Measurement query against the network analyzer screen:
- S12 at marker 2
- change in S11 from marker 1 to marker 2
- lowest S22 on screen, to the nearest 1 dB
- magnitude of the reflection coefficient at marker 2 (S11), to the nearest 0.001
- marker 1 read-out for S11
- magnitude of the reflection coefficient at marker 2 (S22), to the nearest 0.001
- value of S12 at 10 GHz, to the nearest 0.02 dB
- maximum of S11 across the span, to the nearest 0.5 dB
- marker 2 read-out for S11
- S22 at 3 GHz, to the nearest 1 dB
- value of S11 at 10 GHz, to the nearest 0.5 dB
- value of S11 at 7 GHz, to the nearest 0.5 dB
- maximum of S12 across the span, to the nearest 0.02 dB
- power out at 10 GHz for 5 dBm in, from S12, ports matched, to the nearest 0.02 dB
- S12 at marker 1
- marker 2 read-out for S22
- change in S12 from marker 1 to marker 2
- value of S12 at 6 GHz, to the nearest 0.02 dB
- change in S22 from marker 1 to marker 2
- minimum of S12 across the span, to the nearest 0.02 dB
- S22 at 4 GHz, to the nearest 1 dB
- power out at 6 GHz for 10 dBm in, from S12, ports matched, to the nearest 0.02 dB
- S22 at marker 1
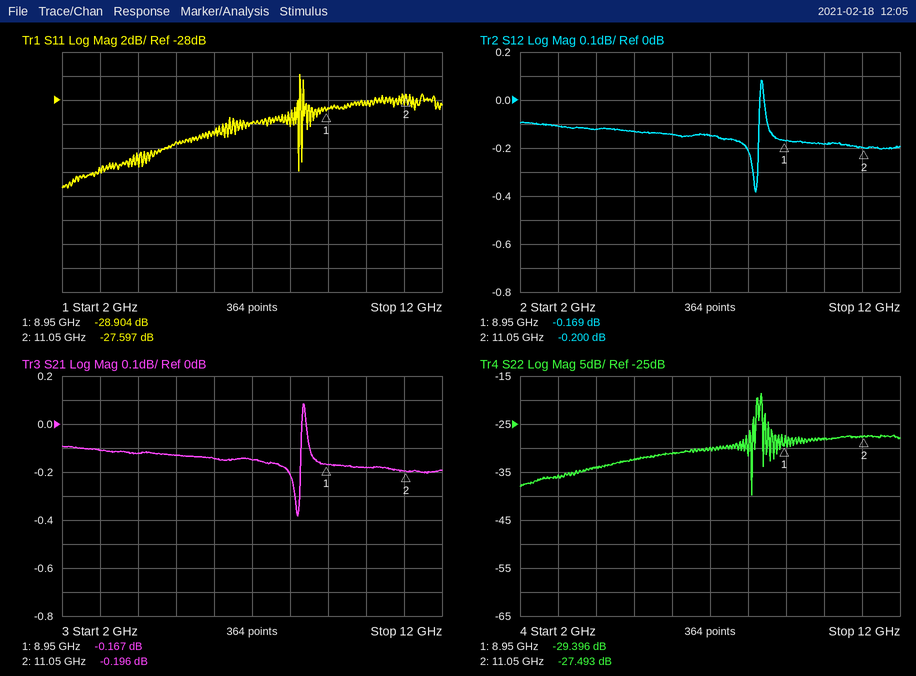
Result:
-0.200 dB
1.307 dB
-40 dB
0.042
-28.904 dB
0.042
-0.18 dB
-26.0 dB
-27.597 dB
-36 dB
-28.5 dB
-30.0 dB
0.08 dB
4.82 dBm
-0.169 dB
-27.493 dB
-0.031 dB
-0.14 dB
1.903 dB
-0.38 dB
-34 dB
9.86 dBm
-29.396 dB
